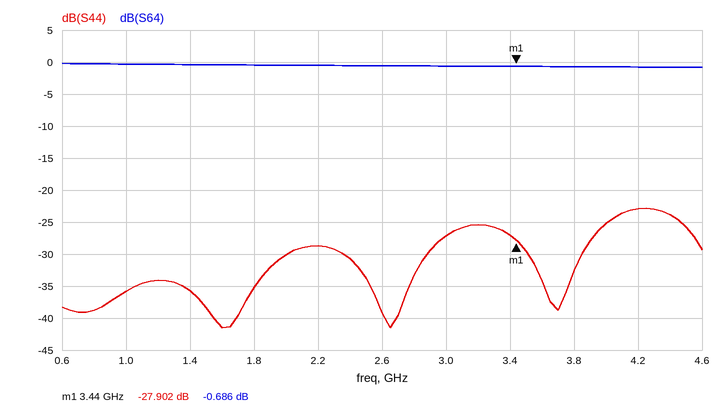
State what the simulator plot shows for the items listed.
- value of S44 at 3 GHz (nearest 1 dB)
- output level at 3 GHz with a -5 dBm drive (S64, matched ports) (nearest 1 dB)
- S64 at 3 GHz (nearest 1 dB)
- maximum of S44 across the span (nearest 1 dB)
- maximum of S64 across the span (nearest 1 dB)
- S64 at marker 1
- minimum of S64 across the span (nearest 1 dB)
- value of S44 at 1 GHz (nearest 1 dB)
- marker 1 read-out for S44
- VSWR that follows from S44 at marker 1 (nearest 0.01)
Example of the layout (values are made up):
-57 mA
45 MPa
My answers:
-27 dB
-6 dBm
-1 dB
-23 dB
0 dB
-0.686 dB
-1 dB
-36 dB
-27.902 dB
1.08
